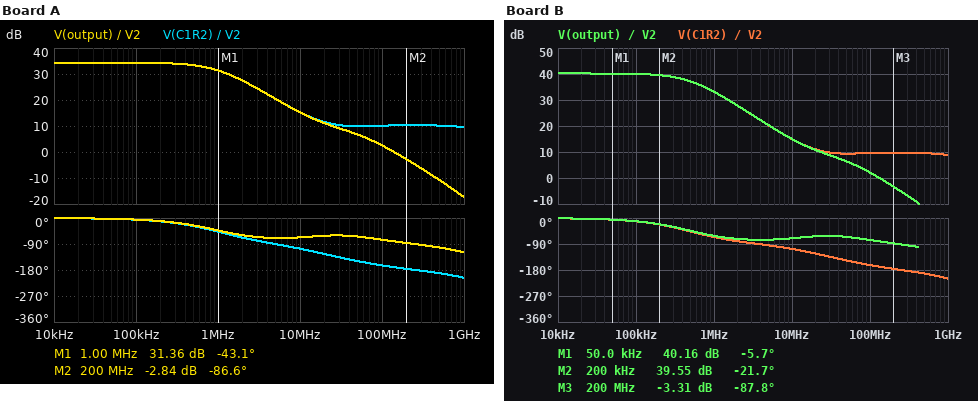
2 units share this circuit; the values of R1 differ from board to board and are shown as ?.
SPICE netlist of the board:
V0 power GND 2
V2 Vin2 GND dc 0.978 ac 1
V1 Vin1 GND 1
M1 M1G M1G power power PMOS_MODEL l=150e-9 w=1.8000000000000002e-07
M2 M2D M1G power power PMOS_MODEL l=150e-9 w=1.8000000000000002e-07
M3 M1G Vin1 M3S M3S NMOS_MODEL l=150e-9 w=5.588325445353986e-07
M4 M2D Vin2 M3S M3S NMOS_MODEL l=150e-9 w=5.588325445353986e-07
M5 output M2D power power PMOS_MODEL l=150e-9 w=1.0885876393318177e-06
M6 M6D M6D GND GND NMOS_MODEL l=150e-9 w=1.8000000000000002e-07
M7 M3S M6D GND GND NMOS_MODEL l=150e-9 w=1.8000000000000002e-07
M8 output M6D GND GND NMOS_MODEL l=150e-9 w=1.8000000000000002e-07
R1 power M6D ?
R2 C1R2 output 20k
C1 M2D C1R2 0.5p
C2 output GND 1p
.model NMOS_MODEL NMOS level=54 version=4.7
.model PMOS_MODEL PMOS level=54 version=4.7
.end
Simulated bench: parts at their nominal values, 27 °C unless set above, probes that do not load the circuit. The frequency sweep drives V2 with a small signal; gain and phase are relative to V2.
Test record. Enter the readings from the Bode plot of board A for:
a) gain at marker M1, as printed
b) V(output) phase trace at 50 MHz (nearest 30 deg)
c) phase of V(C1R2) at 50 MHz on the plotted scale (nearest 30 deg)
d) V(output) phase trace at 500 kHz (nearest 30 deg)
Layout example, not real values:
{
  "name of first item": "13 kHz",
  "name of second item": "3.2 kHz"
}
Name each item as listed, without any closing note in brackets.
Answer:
{
  "gain at marker M1, as printed": "31.36 dB",
  "V(output) phase trace at 50 MHz": "-60 deg",
  "phase of V(C1R2) at 50 MHz on the plotted scale": "-150 deg",
  "V(output) phase trace at 500 kHz": "-30 deg"
}
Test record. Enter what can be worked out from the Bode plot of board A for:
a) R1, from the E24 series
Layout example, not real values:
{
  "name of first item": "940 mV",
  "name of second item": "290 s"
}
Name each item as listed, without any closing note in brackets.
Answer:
{
  "R1, from the E24 series": "11 kΩ"
}
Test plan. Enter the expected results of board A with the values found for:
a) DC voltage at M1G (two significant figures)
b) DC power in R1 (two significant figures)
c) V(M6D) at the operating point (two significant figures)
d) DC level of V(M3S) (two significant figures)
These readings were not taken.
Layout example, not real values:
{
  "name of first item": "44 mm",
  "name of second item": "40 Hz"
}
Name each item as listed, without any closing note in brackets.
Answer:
{
  "DC voltage at M1G": "1.0 V",
  "DC power in R1": "73 µW",
  "V(M6D) at the operating point": "1.1 V",
  "DC level of V(M3S)": "460 mV"
}
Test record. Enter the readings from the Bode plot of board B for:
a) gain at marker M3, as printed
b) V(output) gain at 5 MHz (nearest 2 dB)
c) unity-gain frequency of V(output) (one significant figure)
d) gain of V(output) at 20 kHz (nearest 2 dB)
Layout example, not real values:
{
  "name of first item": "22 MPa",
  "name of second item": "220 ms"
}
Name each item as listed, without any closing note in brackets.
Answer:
{
  "gain at marker M3, as printed": "-3.31 dB",
  "V(output) gain at 5 MHz": "20 dB",
  "unity-gain frequency of V(output)": "100 MHz",
  "gain of V(output) at 20 kHz": "40 dB"
}
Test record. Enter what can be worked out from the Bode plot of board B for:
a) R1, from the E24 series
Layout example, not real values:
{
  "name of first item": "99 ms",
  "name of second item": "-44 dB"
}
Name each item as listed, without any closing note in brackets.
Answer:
{
  "R1, from the E24 series": "27 kΩ"
}
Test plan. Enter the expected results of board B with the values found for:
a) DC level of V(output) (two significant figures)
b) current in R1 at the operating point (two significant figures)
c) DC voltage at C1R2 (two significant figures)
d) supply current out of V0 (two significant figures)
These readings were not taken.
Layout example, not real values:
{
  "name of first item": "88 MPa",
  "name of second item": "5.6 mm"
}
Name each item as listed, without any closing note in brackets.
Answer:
{
  "DC level of V(output)": "390 mV",
  "current in R1 at the operating point": "43 µA",
  "DC voltage at C1R2": "390 mV",
  "supply current out of V0": "120 µA"
}
